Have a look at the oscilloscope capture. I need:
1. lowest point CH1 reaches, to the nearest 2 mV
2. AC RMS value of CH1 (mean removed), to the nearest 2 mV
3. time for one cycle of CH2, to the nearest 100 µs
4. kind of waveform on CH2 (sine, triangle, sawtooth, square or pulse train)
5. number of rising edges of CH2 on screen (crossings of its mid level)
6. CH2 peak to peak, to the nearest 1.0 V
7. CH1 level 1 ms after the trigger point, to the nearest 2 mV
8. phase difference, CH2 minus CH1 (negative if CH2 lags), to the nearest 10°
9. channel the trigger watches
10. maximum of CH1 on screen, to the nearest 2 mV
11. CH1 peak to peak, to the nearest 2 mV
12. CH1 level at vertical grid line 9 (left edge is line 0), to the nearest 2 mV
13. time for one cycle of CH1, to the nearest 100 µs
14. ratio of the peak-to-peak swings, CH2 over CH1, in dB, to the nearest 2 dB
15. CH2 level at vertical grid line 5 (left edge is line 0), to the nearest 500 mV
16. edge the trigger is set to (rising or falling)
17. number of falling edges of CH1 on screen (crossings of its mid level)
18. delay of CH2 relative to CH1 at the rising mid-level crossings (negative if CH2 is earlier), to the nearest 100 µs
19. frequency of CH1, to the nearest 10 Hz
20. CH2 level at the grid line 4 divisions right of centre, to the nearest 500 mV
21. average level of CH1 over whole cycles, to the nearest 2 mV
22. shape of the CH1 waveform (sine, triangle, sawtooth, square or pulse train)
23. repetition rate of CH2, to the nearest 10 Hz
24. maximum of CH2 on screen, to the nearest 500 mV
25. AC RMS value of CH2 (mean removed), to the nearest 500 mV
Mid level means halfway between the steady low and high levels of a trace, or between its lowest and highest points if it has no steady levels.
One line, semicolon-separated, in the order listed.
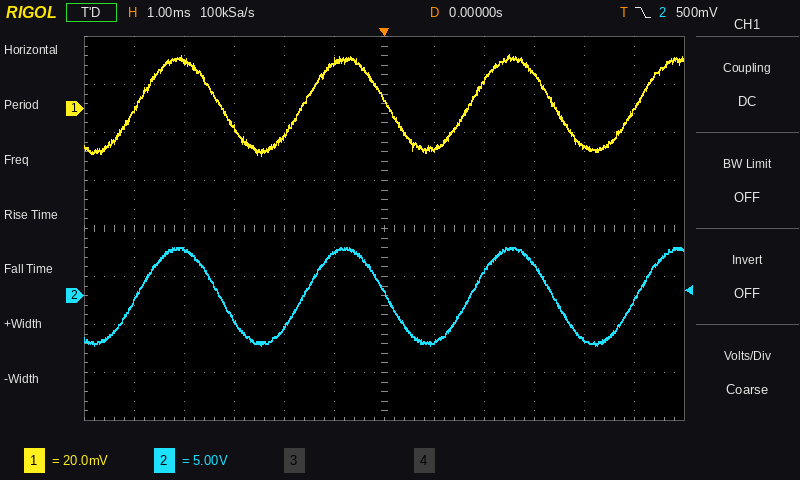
-20 mV; 14 mV; 3.3 ms; sine; 4; 10.0 V; -16 mV; 0°; CH2; 22 mV; 42 mV; 14 mV; 3.3 ms; 48 dB; 4.5 V; falling; 3; 0.0 ms; 300 Hz; -4.5 V; 2 mV; sine; 300 Hz; 5.0 V; 3.5 V
